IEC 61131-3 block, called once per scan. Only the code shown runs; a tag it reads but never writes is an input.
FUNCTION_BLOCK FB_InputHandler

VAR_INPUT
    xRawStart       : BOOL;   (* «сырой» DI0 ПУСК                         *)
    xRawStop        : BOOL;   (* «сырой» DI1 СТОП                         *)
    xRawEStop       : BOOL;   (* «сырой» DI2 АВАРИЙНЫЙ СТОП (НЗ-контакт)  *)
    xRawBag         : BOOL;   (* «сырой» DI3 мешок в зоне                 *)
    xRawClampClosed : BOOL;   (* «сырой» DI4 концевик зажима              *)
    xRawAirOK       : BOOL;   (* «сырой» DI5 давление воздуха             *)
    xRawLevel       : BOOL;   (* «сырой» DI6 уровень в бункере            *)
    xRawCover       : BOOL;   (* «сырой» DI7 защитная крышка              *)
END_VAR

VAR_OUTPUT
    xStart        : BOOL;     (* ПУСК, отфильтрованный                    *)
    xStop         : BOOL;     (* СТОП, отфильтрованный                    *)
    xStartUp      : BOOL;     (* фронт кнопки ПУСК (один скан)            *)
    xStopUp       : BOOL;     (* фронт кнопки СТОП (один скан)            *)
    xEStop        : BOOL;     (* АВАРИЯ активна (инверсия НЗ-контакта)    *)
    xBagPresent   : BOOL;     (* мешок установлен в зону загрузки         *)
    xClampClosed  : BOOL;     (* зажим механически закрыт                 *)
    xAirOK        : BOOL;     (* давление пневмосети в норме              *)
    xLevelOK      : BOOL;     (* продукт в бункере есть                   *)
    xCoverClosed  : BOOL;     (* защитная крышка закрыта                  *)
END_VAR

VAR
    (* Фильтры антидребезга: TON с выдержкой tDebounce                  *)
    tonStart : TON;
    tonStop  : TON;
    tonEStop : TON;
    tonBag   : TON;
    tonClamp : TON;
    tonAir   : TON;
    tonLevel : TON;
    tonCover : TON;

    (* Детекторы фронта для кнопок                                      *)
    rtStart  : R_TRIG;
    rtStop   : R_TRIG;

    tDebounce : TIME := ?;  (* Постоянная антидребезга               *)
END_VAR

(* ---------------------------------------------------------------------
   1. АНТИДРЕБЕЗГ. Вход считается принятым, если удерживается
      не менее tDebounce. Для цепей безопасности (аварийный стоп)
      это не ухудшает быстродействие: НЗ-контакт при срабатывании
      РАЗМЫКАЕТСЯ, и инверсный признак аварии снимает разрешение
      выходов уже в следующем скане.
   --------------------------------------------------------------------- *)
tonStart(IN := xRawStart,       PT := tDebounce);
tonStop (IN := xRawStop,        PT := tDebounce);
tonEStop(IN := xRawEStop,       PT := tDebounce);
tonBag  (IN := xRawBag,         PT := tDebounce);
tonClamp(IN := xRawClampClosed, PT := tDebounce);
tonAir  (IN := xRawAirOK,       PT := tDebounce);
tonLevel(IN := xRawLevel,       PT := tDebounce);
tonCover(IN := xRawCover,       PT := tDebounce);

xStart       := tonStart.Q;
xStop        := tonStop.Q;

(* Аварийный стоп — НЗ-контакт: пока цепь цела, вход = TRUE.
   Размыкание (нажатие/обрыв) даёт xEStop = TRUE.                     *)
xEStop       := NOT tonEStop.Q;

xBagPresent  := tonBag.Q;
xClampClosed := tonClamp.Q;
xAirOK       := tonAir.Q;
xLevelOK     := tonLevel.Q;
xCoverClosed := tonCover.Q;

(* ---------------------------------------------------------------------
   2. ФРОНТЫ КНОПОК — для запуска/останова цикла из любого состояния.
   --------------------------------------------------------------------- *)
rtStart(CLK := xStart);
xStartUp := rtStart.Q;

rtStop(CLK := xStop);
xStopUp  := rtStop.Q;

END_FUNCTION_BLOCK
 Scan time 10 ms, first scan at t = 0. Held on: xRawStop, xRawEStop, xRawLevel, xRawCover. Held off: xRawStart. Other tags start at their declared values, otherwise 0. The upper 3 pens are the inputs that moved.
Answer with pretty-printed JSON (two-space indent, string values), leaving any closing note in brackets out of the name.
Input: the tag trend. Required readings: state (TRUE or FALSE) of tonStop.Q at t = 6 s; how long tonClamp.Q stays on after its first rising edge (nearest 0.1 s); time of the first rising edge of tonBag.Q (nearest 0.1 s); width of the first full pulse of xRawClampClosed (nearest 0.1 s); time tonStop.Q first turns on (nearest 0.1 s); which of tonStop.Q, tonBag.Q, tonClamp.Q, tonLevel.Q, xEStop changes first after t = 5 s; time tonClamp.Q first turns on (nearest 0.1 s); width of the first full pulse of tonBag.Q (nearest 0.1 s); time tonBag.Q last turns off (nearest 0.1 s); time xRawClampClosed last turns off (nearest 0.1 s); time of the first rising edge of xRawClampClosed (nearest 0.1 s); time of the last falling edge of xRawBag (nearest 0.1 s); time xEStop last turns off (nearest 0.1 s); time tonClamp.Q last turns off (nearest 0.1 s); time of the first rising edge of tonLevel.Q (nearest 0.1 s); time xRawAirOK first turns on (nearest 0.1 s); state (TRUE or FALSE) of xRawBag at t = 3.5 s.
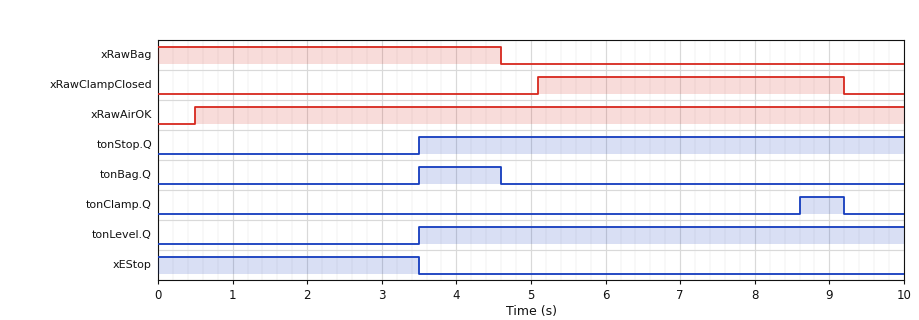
{
  "state (TRUE or FALSE) of tonStop.Q at t = 6 s": "TRUE",
  "how long tonClamp.Q stays on after its first rising edge": "0.6 s",
  "time of the first rising edge of tonBag.Q": "3.5 s",
  "width of the first full pulse of xRawClampClosed": "4.1 s",
  "time tonStop.Q first turns on": "3.5 s",
  "which of tonStop.Q, tonBag.Q, tonClamp.Q, tonLevel.Q, xEStop changes first after t = 5 s": "tonClamp.Q",
  "time tonClamp.Q first turns on": "8.6 s",
  "width of the first full pulse of tonBag.Q": "1.1 s",
  "time tonBag.Q last turns off": "4.6 s",
  "time xRawClampClosed last turns off": "9.2 s",
  "time of the first rising edge of xRawClampClosed": "5.1 s",
  "time of the last falling edge of xRawBag": "4.6 s",
  "time xEStop last turns off": "3.5 s",
  "time tonClamp.Q last turns off": "9.2 s",
  "time of the first rising edge of tonLevel.Q": "3.5 s",
  "time xRawAirOK first turns on": "0.5 s",
  "state (TRUE or FALSE) of xRawBag at t = 3.5 s": "TRUE"
}
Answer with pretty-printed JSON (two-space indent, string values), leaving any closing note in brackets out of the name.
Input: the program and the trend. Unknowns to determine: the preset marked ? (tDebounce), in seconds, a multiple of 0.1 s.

{
  "the preset marked ? (tDebounce), in seconds, a multiple of 0.1 s": "3.5 s"
}
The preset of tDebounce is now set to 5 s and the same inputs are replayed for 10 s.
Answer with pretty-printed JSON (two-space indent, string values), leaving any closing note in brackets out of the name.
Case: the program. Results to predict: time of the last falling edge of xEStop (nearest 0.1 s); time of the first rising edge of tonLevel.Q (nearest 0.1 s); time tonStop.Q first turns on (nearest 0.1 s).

{
  "time of the last falling edge of xEStop": "5.0 s",
  "time of the first rising edge of tonLevel.Q": "5.0 s",
  "time tonStop.Q first turns on": "5.0 s"
}
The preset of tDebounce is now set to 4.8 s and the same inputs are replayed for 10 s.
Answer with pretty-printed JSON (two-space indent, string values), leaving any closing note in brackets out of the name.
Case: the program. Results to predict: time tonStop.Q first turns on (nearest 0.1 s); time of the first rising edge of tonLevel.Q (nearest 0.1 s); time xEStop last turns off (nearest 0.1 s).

{
  "time tonStop.Q first turns on": "4.8 s",
  "time of the first rising edge of tonLevel.Q": "4.8 s",
  "time xEStop last turns off": "4.8 s"
}
